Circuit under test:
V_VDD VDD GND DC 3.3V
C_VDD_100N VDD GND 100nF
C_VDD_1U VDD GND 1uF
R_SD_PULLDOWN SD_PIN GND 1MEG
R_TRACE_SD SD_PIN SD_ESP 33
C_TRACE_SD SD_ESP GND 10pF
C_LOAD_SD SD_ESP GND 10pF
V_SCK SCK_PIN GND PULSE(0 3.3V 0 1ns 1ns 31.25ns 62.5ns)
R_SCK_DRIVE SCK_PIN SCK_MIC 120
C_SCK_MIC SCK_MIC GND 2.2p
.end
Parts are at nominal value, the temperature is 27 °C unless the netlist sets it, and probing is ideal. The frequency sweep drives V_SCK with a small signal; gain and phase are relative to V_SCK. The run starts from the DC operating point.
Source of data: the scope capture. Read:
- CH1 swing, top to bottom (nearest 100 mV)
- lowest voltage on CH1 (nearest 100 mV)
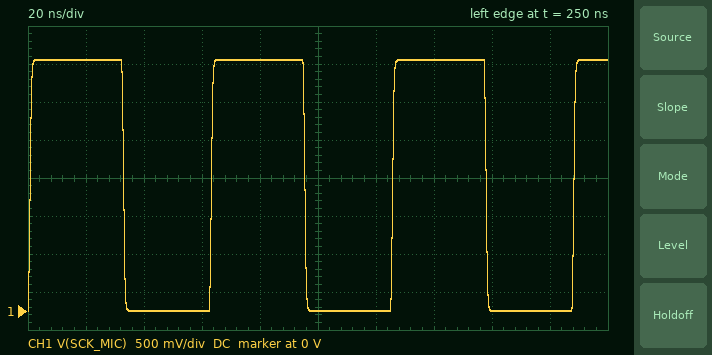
3.3 V
0 V
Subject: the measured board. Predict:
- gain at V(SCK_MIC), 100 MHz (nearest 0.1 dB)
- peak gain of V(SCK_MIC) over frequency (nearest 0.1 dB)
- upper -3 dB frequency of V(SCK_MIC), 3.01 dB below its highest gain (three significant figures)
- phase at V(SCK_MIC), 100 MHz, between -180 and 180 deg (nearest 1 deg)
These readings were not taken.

-0.1 dB
0 dB
603 MHz
-9 deg
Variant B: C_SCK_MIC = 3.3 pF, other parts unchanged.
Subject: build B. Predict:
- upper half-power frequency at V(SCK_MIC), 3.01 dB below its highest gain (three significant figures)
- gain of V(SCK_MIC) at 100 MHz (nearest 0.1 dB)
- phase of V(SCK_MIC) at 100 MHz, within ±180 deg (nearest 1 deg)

402 MHz
-0.3 dB
-14 deg
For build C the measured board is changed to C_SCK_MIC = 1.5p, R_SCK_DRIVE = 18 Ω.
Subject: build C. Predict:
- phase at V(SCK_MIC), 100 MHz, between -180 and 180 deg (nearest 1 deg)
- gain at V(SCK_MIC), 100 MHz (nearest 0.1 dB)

-1 deg
0 dB
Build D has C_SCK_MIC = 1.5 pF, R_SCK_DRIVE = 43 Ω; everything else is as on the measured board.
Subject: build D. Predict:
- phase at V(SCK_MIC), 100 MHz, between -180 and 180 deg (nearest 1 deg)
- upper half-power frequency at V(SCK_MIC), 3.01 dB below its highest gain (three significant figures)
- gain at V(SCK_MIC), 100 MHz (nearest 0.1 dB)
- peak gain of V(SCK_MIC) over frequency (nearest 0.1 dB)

-2 deg
2.47 GHz
0 dB
0 dB
